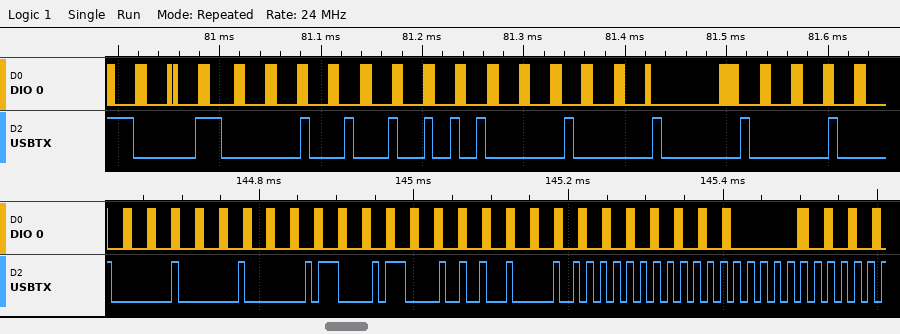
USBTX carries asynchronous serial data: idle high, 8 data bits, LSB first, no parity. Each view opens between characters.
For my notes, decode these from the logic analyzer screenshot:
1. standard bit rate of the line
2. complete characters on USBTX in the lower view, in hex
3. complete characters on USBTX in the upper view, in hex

115200 baud
00, 00, 00, 07, 07, 12, 20, 55, 55, 55, 55
C0, 00, 08, 24, 00, 00, 00, 00
